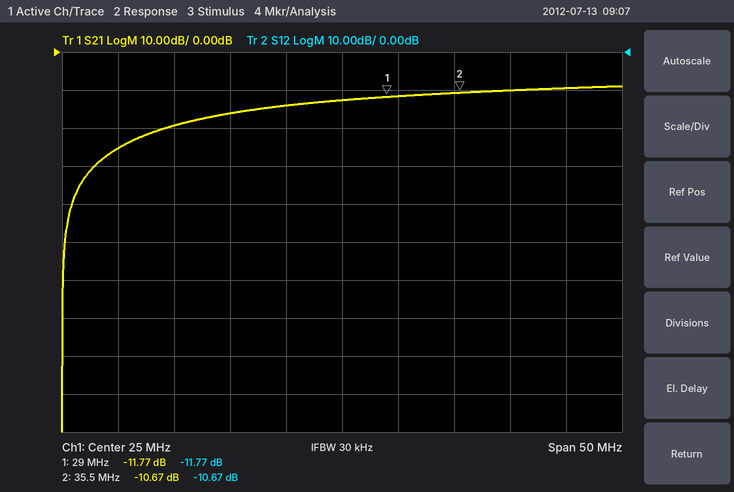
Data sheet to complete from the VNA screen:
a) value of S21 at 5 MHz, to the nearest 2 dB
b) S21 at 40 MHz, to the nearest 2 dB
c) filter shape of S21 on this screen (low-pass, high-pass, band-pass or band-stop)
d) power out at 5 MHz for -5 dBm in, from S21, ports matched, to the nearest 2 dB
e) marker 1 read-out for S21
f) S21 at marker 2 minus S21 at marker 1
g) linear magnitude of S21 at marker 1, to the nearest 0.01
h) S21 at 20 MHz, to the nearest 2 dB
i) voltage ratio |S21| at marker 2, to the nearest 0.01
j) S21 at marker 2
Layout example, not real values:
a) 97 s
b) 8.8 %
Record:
a) -26 dB
b) -10 dB
c) high-pass
d) -30 dBm
e) -11.77 dB
f) 1.10 dB
g) 0.26
h) -14 dB
i) 0.29
j) -10.67 dB
